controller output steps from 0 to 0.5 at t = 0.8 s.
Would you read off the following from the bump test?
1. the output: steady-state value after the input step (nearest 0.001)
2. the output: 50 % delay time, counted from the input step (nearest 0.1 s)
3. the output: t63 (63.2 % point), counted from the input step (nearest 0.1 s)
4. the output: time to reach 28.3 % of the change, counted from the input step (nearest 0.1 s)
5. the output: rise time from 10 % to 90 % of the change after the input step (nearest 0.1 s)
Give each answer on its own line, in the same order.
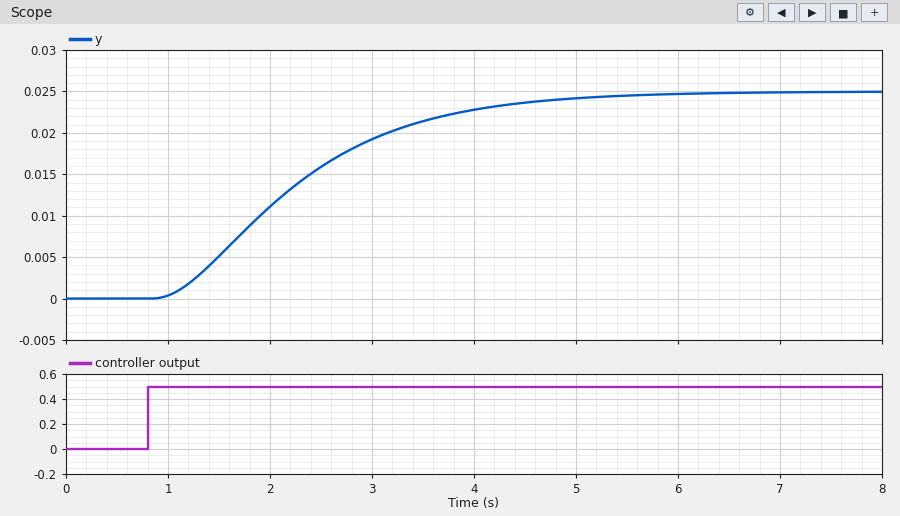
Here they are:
0.025
1.3 s
1.7 s
0.9 s
2.6 s
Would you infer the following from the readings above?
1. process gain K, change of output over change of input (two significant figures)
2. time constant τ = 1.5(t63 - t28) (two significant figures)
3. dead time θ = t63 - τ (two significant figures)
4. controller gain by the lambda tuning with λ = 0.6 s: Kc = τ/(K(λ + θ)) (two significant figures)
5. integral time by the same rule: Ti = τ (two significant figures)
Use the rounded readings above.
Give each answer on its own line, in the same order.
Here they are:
0.050
1.2 s
0.50 s
22
1.2 s
